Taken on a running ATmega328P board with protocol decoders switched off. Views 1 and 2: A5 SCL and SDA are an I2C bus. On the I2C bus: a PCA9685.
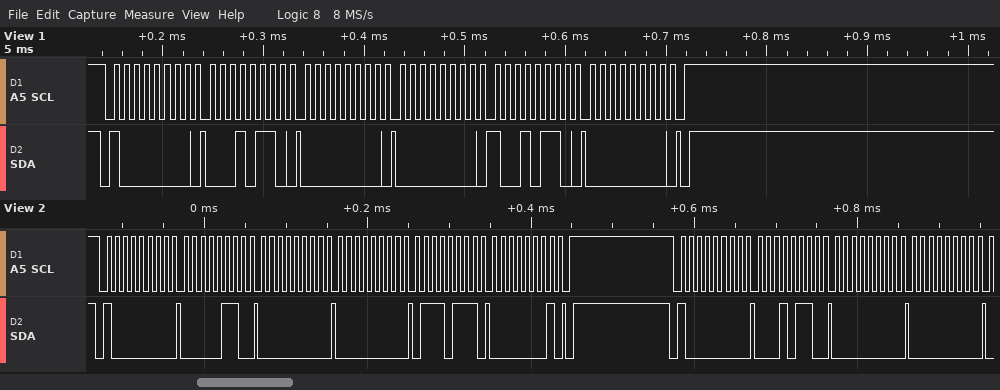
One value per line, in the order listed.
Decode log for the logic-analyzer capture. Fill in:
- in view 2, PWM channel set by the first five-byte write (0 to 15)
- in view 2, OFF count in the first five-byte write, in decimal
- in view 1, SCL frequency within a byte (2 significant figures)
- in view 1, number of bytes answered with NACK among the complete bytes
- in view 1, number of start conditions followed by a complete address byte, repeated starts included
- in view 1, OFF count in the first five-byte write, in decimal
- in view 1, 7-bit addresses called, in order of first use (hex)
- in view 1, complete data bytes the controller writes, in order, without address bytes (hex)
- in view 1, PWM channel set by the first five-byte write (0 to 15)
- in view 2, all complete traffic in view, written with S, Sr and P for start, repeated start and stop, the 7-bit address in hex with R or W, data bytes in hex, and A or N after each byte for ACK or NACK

0
375
100 kHz
0
1
150
0x40
16 00 00 96 00
4
S 40W A 06 A 00 A 00 A 77 A 01 A P S 40W A 16 A 00 A 00 A
